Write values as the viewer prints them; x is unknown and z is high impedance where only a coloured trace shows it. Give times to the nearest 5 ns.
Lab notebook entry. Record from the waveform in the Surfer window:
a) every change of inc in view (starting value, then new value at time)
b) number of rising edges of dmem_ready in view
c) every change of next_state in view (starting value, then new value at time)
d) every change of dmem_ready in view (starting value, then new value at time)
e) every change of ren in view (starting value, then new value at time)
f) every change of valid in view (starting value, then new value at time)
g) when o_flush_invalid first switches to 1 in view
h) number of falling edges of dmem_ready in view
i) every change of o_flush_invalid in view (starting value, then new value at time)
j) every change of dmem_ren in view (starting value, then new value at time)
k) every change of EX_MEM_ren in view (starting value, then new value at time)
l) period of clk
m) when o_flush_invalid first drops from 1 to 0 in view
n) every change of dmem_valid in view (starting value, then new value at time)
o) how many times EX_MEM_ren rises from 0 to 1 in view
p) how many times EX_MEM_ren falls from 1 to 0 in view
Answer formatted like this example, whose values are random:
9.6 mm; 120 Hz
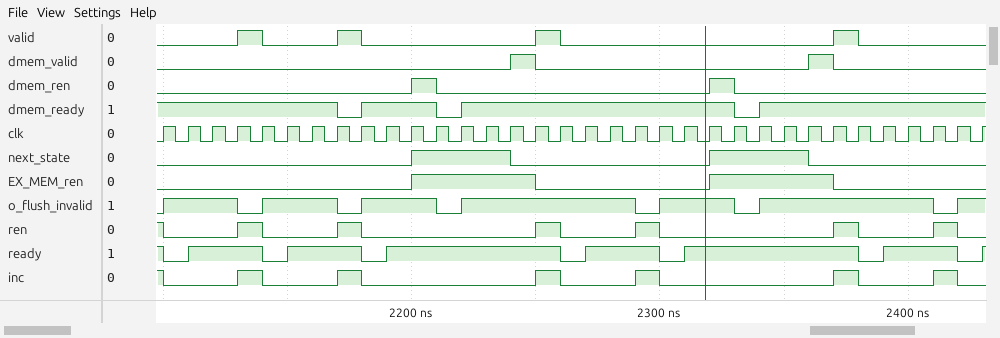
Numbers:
1, 0 at 2100 ns, 1 at 2130 ns, 0 at 2140 ns, 1 at 2170 ns, 0 at 2180 ns, 1 at 2250 ns, 0 at 2260 ns, 1 at 2290 ns, 0 at 2300 ns, 1 at 2370 ns, 0 at 2380 ns, 1 at 2410 ns, 0 at 2420 ns; 3; 0, 1 at 2200 ns, 0 at 2240 ns, 1 at 2320 ns, 0 at 2360 ns; 1, 0 at 2170 ns, 1 at 2180 ns, 0 at 2210 ns, 1 at 2220 ns, 0 at 2330 ns, 1 at 2340 ns; 1, 0 at 2100 ns, 1 at 2130 ns, 0 at 2140 ns, 1 at 2170 ns, 0 at 2180 ns, 1 at 2250 ns, 0 at 2260 ns, 1 at 2290 ns, 0 at 2300 ns, 1 at 2370 ns, 0 at 2380 ns, 1 at 2410 ns, 0 at 2420 ns; 0, 1 at 2130 ns, 0 at 2140 ns, 1 at 2170 ns, 0 at 2180 ns, 1 at 2250 ns, 0 at 2260 ns, 1 at 2370 ns, 0 at 2380 ns; 2100 ns; 3; 0, 1 at 2100 ns, 0 at 2130 ns, 1 at 2140 ns, 0 at 2170 ns, 1 at 2180 ns, 0 at 2210 ns, 1 at 2220 ns, 0 at 2290 ns, 1 at 2300 ns, 0 at 2330 ns, 1 at 2340 ns, 0 at 2410 ns, 1 at 2420 ns; 0, 1 at 2200 ns, 0 at 2210 ns, 1 at 2320 ns, 0 at 2330 ns; 0, 1 at 2200 ns, 0 at 2250 ns, 1 at 2320 ns, 0 at 2370 ns; 10 ns; 2130 ns; 0, 1 at 2240 ns, 0 at 2250 ns, 1 at 2360 ns, 0 at 2370 ns; 2; 2
